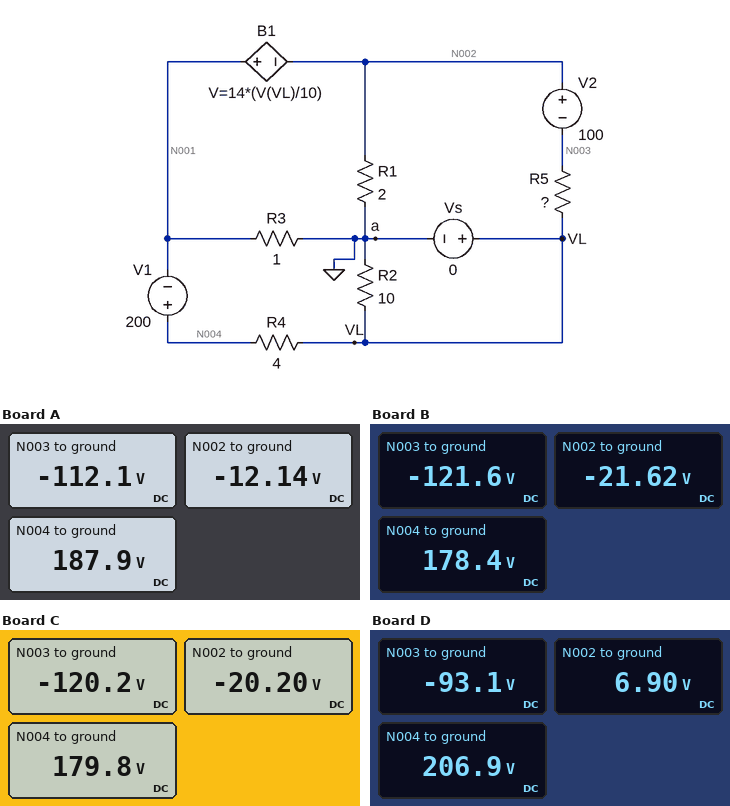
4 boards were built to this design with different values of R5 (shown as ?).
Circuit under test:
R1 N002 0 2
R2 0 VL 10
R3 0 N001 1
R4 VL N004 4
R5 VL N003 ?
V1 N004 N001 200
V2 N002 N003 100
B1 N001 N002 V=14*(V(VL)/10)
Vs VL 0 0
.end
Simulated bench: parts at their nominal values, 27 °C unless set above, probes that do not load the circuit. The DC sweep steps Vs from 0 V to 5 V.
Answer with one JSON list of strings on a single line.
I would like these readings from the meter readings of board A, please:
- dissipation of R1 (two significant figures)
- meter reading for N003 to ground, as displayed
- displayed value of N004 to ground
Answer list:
["74 W", "-112.1 V", "187.9 V"]
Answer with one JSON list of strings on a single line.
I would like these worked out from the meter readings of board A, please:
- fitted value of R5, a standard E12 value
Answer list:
["3.9 Ω"]
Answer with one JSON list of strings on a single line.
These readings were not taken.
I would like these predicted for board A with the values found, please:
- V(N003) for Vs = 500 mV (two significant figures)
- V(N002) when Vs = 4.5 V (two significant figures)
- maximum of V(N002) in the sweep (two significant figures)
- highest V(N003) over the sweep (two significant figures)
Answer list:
["-110 V", "-15 V", "-12 V", "-110 V"]
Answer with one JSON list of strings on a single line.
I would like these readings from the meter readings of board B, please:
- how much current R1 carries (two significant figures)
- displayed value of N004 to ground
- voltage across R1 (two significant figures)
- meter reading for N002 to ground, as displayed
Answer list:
["11 A", "178.4 V", "22 V", "-21.62 V"]
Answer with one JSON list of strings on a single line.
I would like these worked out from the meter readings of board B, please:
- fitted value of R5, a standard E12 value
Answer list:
["10 Ω"]
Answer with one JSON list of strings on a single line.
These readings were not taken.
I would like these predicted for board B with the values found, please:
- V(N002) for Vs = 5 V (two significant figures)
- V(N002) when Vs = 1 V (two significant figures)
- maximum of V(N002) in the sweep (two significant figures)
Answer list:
["-25 V", "-22 V", "-22 V"]
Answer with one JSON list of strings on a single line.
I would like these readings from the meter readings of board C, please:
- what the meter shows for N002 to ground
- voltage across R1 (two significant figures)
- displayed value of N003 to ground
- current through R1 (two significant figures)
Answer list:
["-20.20 V", "20 V", "-120.2 V", "10 A"]
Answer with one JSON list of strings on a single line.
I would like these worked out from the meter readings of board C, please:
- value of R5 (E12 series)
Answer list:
["8.2 Ω"]
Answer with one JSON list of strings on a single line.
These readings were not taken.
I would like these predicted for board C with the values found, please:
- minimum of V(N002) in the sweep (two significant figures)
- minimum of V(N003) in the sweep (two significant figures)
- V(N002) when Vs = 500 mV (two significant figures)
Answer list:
["-24 V", "-120 V", "-21 V"]
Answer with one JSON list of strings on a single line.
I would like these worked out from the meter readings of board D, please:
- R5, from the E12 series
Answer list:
["1.5 Ω"]
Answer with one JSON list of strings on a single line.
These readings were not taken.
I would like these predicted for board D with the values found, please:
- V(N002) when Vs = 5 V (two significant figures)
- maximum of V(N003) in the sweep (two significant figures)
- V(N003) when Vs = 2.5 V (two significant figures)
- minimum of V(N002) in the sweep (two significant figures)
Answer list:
["5.2 V", "-93 V", "-94 V", "5.2 V"]
